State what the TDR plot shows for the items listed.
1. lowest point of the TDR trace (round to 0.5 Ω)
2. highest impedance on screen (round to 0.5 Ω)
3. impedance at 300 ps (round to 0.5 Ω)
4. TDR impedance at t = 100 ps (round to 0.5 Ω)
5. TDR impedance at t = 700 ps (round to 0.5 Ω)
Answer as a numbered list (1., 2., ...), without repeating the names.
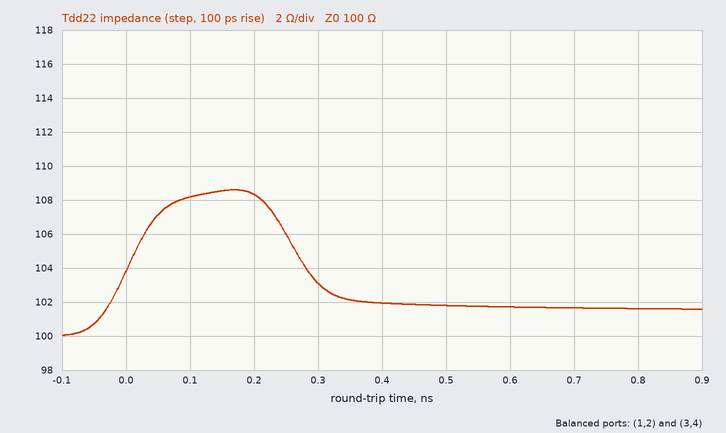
1. 100.0 Ω
2. 108.5 Ω
3. 103.0 Ω
4. 108.0 Ω
5. 101.5 Ω
